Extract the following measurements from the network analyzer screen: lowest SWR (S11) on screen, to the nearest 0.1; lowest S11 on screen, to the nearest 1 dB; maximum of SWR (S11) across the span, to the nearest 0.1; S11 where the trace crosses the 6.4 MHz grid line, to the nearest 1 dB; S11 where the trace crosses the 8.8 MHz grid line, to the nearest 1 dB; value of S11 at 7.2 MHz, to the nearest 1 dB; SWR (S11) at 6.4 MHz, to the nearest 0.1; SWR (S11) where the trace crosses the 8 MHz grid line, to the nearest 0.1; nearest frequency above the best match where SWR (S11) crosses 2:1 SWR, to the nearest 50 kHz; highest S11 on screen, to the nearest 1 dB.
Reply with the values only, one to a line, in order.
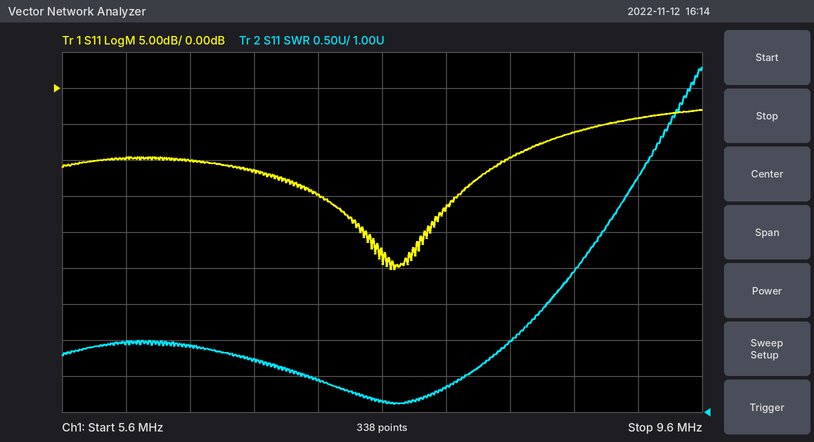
1.1
-25 dB
5.8
-10 dB
-6 dB
-15 dB
1.9
1.3
8.40 MHz
-3 dB
